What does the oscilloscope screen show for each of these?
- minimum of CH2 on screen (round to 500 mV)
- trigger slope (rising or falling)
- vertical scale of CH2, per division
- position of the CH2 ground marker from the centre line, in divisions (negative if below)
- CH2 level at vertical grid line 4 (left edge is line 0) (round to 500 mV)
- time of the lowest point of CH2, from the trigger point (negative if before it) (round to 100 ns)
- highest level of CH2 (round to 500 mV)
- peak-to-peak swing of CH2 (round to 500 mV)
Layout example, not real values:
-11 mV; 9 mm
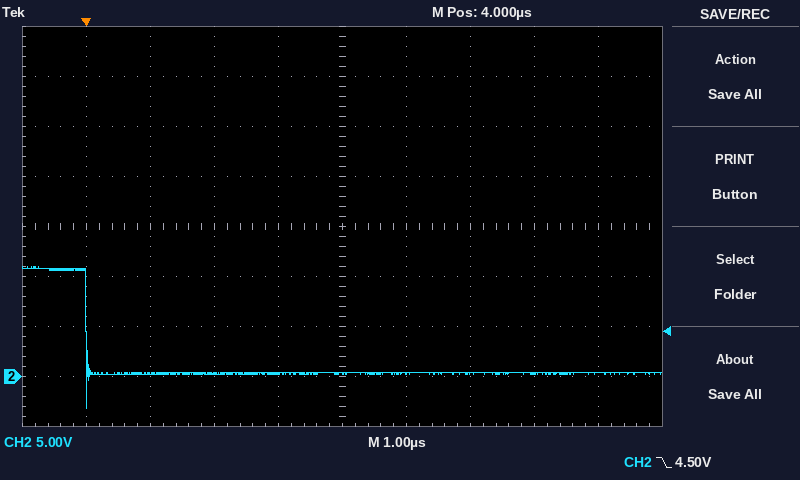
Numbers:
-3.0 V; falling; 5 V; -3.0 div; 500 mV; 0.0 µs; 11.0 V; 14.0 V
